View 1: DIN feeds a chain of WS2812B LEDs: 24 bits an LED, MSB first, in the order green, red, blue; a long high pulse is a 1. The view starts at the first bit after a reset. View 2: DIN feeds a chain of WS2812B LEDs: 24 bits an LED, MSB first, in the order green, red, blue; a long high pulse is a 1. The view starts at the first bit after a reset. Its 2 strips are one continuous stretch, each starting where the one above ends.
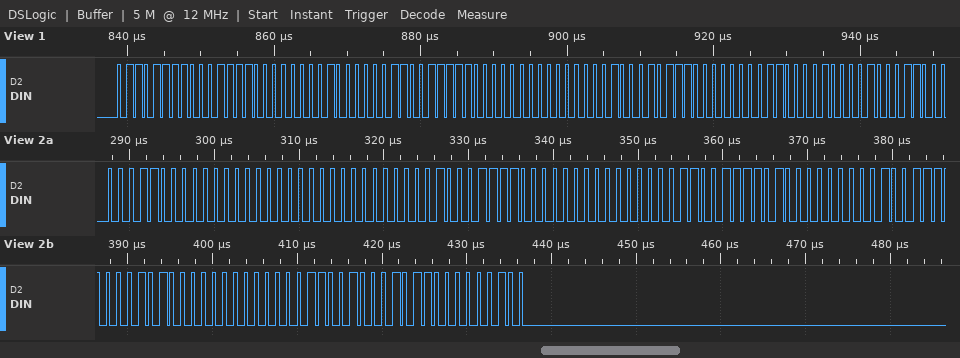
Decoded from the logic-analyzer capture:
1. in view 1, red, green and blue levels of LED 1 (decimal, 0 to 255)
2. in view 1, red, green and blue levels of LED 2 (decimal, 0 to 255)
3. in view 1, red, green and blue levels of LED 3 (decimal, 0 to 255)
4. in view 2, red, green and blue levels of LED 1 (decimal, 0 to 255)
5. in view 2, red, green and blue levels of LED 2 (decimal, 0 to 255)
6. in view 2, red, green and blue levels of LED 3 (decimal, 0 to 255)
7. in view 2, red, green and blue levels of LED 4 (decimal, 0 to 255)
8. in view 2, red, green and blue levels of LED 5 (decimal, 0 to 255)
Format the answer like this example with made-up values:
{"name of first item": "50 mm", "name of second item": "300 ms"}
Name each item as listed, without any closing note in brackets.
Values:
{"in view 1, red, green and blue levels of LED 1": "30, 111, 1", "in view 1, red, green and blue levels of LED 2": "62, 3, 0", "in view 1, red, green and blue levels of LED 3": "46, 2, 1", "in view 2, red, green and blue levels of LED 1": "0, 24, 0", "in view 2, red, green and blue levels of LED 2": "30, 1, 0", "in view 2, red, green and blue levels of LED 3": "61, 3, 0", "in view 2, red, green and blue levels of LED 4": "20, 78, 0", "in view 2, red, green and blue levels of LED 5": "22, 25, 4"}
